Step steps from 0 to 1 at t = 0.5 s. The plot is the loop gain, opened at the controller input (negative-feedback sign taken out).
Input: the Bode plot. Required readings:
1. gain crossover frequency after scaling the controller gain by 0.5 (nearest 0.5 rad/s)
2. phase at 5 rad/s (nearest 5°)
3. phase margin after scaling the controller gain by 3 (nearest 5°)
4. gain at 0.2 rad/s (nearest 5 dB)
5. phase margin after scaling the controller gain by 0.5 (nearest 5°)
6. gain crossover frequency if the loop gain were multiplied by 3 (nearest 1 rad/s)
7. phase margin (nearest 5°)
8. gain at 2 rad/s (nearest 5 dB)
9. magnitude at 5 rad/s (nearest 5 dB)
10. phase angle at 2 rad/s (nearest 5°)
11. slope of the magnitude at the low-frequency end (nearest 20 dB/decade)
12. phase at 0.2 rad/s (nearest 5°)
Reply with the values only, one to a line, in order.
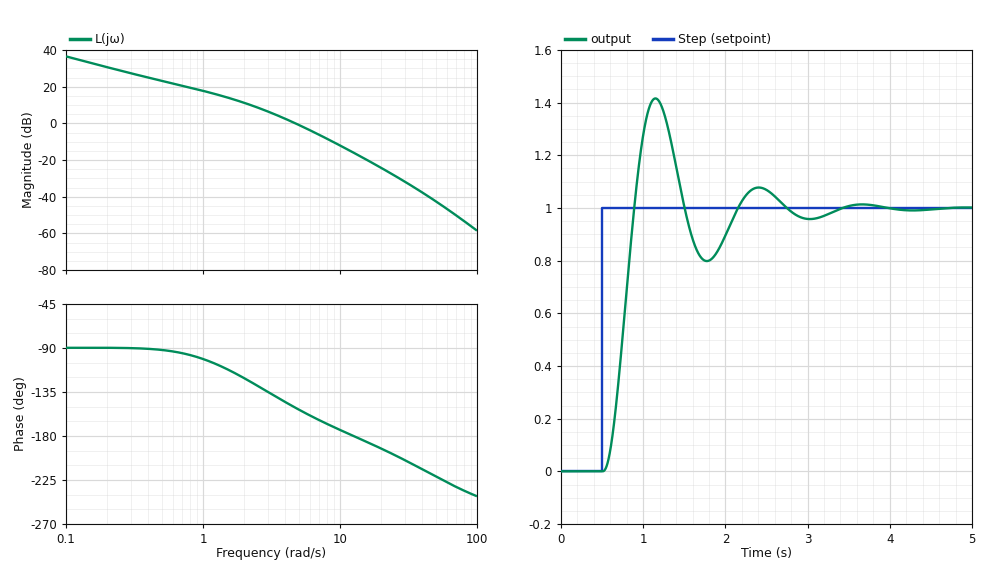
3.0 rad/s
-155°
10°
30 dB
45°
9 rad/s
30°
10 dB
0 dB
-120°
-20 dB/decade
-90°
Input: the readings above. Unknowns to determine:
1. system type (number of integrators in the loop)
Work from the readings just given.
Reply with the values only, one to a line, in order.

1
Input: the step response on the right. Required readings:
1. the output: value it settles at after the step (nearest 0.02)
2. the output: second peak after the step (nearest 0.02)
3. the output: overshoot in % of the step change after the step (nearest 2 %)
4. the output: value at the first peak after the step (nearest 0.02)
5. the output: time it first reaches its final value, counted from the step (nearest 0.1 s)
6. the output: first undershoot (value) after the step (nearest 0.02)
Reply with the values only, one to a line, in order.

1.00
1.08
42 %
1.42
0.4 s
0.80
